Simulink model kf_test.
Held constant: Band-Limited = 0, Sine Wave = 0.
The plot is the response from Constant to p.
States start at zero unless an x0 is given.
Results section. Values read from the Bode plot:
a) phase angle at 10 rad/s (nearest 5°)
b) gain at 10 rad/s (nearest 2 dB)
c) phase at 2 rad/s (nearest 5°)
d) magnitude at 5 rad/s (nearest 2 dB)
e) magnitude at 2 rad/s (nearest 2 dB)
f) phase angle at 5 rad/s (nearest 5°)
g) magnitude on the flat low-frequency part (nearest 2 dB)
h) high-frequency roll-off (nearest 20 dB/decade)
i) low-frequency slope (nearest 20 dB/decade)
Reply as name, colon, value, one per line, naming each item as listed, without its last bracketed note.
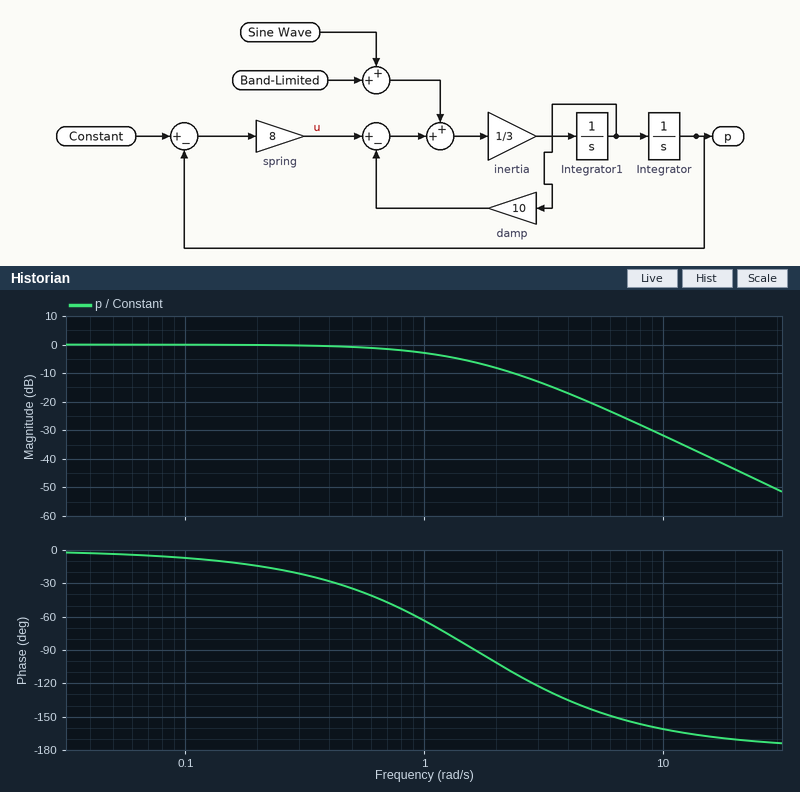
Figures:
phase angle at 10 rad/s: -160°
gain at 10 rad/s: -32 dB
phase at 2 rad/s: -100°
magnitude at 5 rad/s: -20 dB
magnitude at 2 rad/s: -8 dB
phase angle at 5 rad/s: -145°
magnitude on the flat low-frequency part: 0 dB
high-frequency roll-off: -40 dB/decade
low-frequency slope: 0 dB/decade
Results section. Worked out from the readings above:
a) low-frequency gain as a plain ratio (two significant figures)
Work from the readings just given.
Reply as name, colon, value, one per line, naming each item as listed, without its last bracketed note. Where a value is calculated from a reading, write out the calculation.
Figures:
low-frequency gain as a plain ratio: 10^(0 / 20) = 1.0
